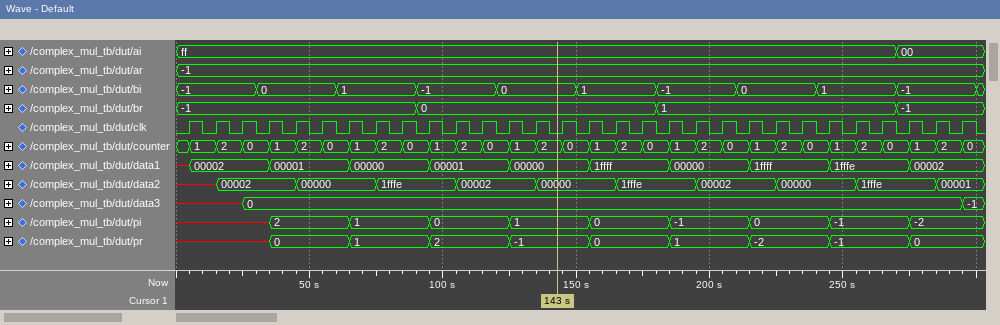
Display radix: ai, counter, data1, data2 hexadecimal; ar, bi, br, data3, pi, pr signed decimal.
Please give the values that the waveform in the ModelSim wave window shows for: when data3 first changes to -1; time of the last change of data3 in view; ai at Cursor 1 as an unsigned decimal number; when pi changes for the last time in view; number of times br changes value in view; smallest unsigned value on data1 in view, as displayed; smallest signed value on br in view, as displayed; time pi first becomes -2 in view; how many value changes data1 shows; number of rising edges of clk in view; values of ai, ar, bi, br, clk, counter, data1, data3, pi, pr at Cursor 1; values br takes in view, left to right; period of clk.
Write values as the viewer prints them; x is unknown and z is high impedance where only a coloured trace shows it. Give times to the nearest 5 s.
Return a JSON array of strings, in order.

["295 s", "295 s", "255", "275 s", "3", "00000", "-1", "275 s", "10", "30", "ai=ff, ar=-1, bi=0, br=0, clk=0, counter=2, data1=00000, data3=0, pi=1, pr=-1", "-1, 0, 1, -1", "10 s"]
